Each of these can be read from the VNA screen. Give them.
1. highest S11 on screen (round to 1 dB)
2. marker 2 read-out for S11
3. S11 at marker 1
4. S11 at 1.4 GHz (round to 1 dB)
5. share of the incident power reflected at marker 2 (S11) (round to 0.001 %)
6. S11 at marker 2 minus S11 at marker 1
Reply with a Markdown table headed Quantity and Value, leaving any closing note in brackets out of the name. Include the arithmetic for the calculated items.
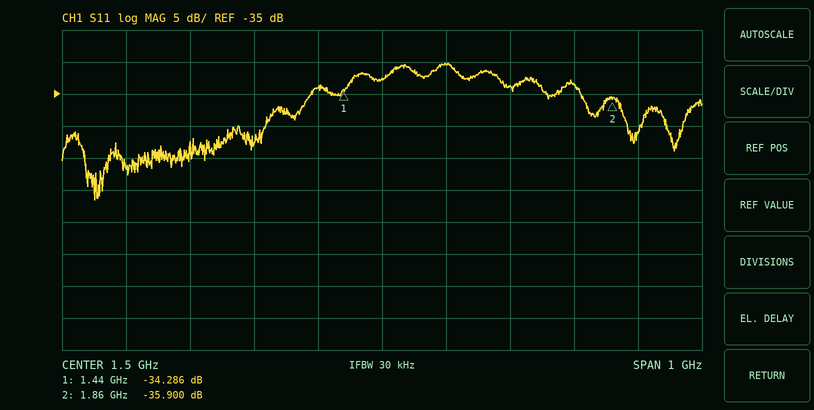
| Quantity | Value |
|---|---|
| highest S11 on screen | -30 dB |
| marker 2 read-out for S11 | -35.900 dB |
| S11 at marker 1 | -34.286 dB |
| S11 at 1.4 GHz | -34 dB |
| share of the incident power reflected at marker 2 (S11) | 10^(-35.9/10) ≈ 0.026 % |
| S11 at marker 2 minus S11 at marker 1 | -35.9 − (-34.286) = -1.614 dB |
